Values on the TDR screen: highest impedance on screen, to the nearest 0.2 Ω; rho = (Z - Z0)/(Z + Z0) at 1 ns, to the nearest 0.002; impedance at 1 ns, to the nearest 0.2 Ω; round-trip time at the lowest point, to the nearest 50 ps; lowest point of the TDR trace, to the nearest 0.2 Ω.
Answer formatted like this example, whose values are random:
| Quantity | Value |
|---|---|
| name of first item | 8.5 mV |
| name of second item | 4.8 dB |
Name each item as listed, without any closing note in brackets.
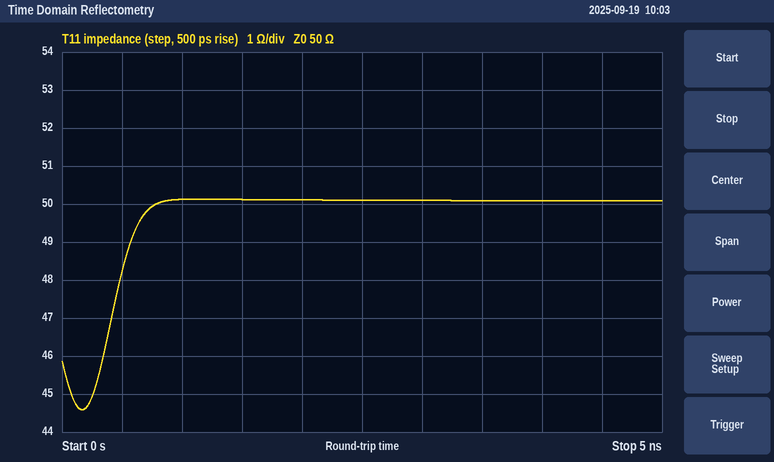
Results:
| Quantity | Value |
|---|---|
| highest impedance on screen, to the nearest 0.2 Ω | 50.2 Ω |
| rho = (Z - Z0)/(Z + Z0) at 1 ns, to the nearest 0.002 | +0.002 |
| impedance at 1 ns, to the nearest 0.2 Ω | 50.2 Ω |
| round-trip time at the lowest point, to the nearest 50 ps | 150 ps |
| lowest point of the TDR trace, to the nearest 0.2 Ω | 44.6 Ω |
